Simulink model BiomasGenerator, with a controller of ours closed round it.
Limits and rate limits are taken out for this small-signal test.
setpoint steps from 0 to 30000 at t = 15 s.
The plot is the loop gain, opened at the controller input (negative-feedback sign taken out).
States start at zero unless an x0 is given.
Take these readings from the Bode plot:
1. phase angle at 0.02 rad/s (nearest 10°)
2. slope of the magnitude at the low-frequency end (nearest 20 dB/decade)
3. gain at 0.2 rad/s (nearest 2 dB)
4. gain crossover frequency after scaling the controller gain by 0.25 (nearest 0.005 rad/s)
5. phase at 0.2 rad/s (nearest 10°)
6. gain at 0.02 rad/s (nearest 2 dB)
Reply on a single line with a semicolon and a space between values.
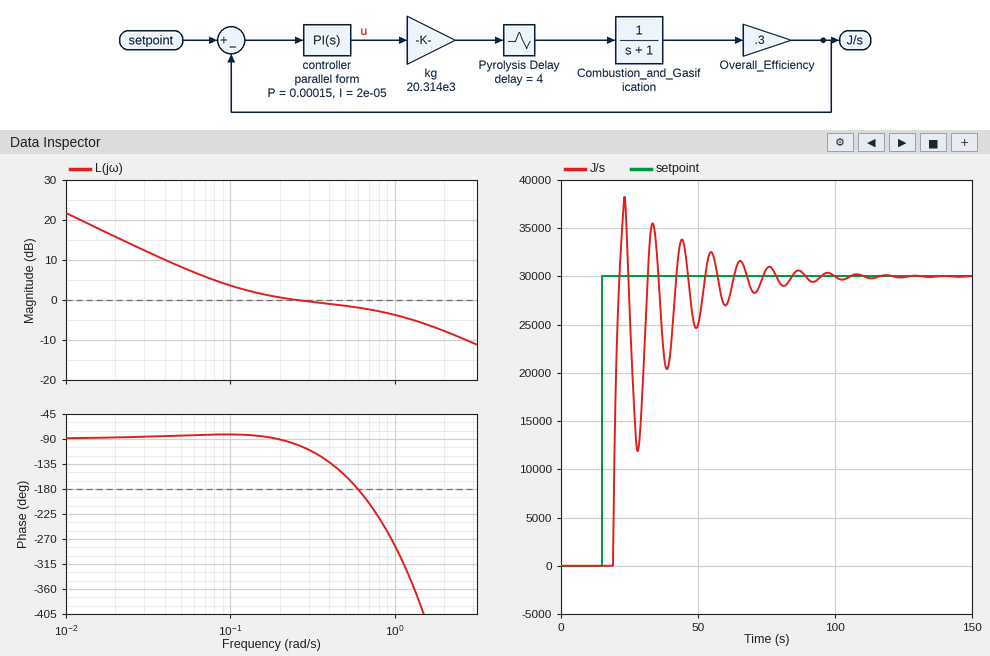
-90°; -20 dB/decade; 0 dB; 0.030 rad/s; -90°; 16 dB
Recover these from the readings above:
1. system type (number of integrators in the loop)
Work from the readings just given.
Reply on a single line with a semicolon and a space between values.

1
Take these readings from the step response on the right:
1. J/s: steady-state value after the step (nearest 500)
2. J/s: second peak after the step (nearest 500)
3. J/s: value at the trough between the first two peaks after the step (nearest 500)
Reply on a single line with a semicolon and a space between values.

30000; 35500; 12000
